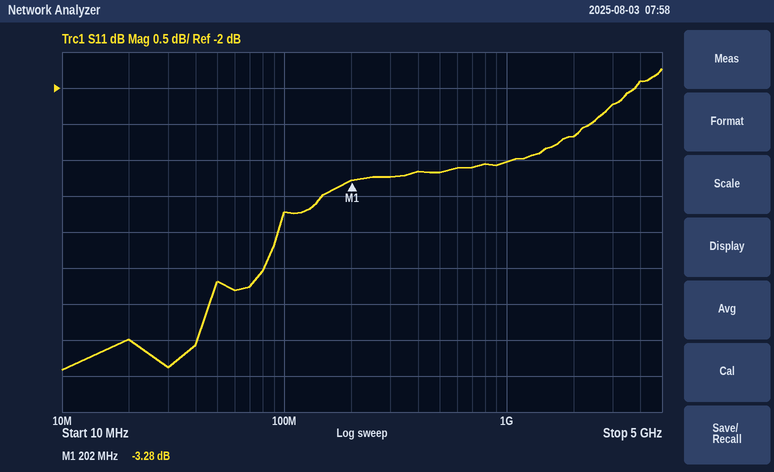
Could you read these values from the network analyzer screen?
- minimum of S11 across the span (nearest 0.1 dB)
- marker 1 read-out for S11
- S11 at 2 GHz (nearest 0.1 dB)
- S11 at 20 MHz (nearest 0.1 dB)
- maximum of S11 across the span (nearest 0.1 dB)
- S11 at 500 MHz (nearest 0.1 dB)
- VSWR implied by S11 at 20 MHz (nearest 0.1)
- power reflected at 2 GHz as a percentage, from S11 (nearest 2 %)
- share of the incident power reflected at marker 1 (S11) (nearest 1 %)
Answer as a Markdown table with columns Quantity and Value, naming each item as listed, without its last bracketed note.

| Quantity | Value |
|---|---|
| minimum of S11 across the span | -5.9 dB |
| marker 1 read-out for S11 | -3.28 dB |
| S11 at 2 GHz | -2.7 dB |
| S11 at 20 MHz | -5.5 dB |
| maximum of S11 across the span | -1.7 dB |
| S11 at 500 MHz | -3.2 dB |
| VSWR implied by S11 at 20 MHz | 3.3 |
| power reflected at 2 GHz as a percentage, from S11 | 54 % |
| share of the incident power reflected at marker 1 (S11) | 47 % |
